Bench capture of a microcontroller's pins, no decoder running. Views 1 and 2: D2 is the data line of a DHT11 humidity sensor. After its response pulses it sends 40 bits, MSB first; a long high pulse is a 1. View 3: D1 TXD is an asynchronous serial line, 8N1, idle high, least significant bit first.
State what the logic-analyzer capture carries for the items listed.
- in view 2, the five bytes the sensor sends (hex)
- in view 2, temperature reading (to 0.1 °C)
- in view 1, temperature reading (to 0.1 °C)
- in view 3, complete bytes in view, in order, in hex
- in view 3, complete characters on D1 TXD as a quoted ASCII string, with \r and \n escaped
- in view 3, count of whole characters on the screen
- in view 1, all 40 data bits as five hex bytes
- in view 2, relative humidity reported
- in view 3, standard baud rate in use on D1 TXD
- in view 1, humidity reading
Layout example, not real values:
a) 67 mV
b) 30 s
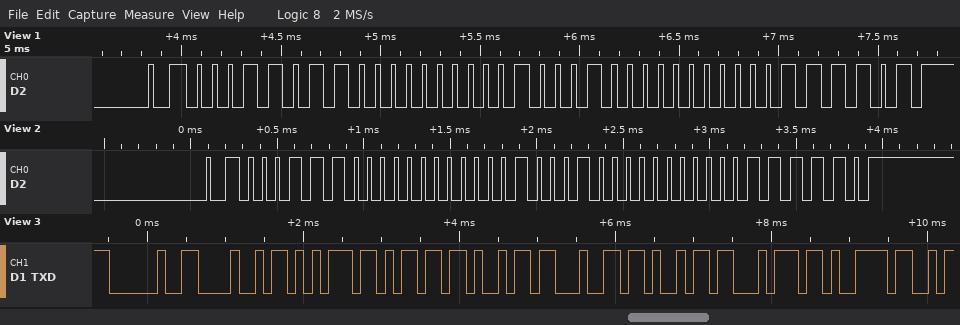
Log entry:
a) 1C 00 22 00 3E
b) 34.0 °C
c) 34.0 °C
d) 20 48 75 6D 69 64 69 74 79
e) " Humidity"
f) 9
g) 1B 00 22 00 3D
h) 28 %
i) 9600 baud
j) 27 %
